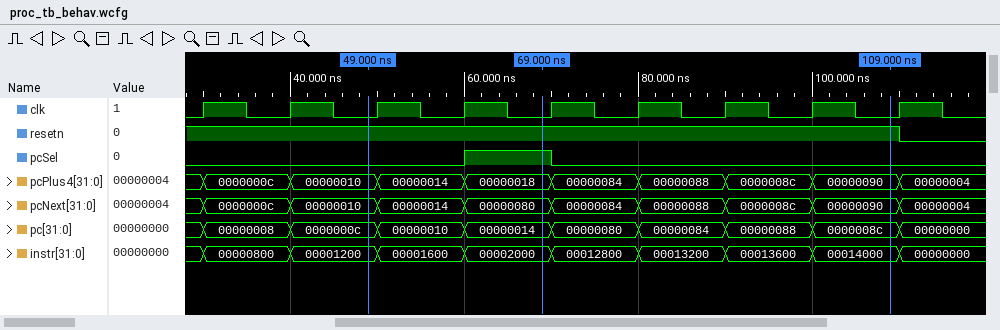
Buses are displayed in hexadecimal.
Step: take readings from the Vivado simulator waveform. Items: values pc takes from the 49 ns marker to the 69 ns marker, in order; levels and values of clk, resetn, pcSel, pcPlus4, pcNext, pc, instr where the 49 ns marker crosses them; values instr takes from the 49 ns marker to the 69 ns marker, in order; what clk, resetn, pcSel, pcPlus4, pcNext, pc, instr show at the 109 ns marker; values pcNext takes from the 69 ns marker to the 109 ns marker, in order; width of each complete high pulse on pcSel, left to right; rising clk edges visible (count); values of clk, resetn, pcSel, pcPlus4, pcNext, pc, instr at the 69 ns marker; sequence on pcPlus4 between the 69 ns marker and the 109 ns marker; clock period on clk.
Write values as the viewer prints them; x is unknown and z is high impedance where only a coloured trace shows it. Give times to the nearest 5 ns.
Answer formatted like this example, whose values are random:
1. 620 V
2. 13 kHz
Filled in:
1. 0000000c, 00000010, 00000014
2. clk=0, resetn=1, pcSel=0, pcPlus4=00000010, pcNext=00000010, pc=0000000c, instr=00001200
3. 00001200, 00001600, 00002000
4. clk=0, resetn=1, pcSel=0, pcPlus4=00000090, pcNext=00000090, pc=0000008c, instr=00014000
5. 00000080, 00000084, 00000088, 0000008c, 00000090
6. 10 ns
7. 9
8. clk=0, resetn=1, pcSel=1, pcPlus4=00000018, pcNext=00000080, pc=00000014, instr=00002000
9. 00000018, 00000084, 00000088, 0000008c, 00000090
10. 10 ns
